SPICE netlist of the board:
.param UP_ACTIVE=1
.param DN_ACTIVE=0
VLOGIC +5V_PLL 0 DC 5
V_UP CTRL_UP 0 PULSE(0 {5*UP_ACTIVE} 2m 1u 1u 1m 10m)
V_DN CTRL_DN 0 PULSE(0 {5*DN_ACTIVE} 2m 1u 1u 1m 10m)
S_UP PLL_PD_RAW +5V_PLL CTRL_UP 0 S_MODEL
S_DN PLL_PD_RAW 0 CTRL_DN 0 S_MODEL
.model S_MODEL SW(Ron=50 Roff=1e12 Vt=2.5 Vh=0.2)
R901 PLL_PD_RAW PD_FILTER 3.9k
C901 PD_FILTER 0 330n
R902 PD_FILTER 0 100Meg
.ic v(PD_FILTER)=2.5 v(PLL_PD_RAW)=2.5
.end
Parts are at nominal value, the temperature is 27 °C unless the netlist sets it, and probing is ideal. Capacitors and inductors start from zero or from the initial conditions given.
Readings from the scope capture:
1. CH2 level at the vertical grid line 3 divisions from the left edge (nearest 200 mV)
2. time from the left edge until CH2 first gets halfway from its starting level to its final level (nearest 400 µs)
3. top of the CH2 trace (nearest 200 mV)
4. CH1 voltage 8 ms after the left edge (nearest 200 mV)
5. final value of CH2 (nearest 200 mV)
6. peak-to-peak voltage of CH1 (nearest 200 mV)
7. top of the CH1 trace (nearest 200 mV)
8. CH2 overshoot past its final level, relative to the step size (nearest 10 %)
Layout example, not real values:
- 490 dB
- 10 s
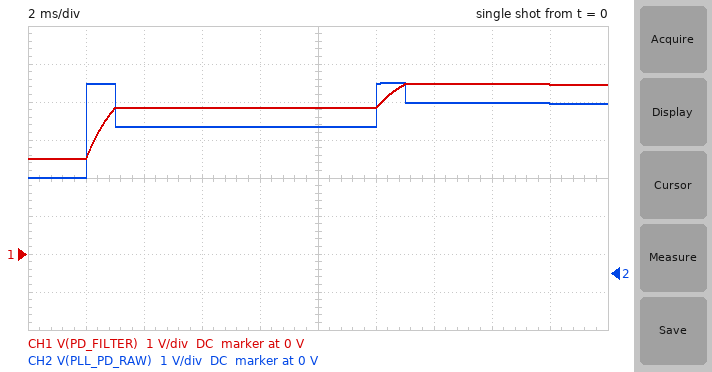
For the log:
- 3.8 V
- 2.0 ms
- 5.0 V
- 3.8 V
- 4.4 V
- 2.0 V
- 4.4 V
- 30 %
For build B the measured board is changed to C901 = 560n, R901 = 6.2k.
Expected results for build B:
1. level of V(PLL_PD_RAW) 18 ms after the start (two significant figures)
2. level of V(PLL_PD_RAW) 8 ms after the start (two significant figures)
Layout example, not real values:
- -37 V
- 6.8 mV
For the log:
- 3.6 V
- 3.1 V
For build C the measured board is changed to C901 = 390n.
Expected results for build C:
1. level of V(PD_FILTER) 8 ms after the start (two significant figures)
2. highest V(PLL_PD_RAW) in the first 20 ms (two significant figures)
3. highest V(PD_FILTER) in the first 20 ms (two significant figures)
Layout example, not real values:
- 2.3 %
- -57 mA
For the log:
- 3.7 V
- 5.0 V
- 4.3 V
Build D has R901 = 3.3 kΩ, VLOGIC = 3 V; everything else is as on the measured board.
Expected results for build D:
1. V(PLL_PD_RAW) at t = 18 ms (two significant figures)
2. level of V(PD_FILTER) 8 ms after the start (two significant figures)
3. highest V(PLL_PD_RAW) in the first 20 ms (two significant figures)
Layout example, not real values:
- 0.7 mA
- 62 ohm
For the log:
- 2.9 V
- 2.8 V
- 3.0 V
